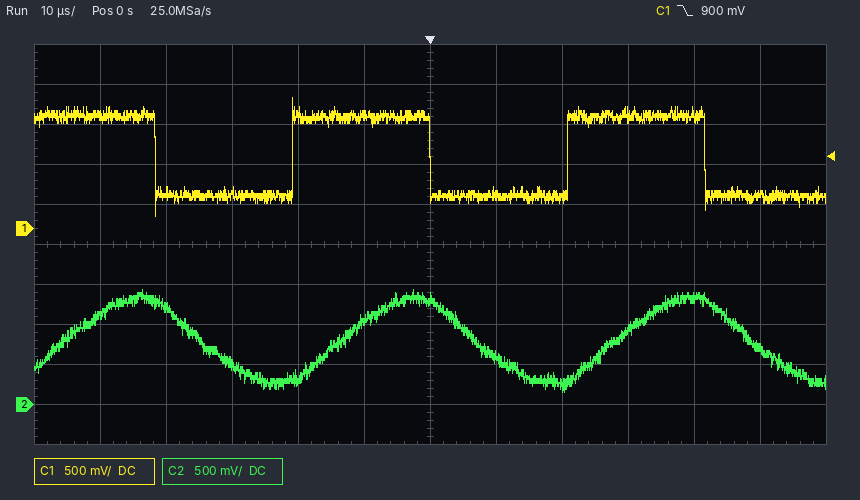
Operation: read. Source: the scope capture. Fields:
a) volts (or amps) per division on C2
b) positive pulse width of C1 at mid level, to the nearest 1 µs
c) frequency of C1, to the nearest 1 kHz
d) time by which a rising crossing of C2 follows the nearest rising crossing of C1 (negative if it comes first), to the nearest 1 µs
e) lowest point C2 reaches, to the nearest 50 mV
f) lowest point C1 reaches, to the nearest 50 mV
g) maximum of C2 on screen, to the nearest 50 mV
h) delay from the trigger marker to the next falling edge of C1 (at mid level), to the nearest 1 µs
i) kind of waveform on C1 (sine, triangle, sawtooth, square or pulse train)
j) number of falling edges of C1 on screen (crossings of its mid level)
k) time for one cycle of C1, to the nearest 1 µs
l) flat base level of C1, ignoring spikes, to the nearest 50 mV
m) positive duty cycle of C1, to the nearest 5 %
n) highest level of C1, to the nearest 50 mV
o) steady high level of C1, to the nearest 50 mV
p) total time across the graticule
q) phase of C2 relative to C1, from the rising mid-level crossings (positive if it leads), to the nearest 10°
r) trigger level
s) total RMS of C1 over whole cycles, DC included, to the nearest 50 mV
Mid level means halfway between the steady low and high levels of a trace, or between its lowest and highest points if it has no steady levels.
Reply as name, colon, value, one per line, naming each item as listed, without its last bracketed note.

volts (or amps) per division on C2: 500 mV
positive pulse width of C1 at mid level, to the nearest 1 µs: 21 µs
frequency of C1, to the nearest 1 kHz: 24 kHz
time by which a rising crossing of C2 follows the nearest rising crossing of C1 (negative if it comes first), to the nearest 1 µs: +7 µs
lowest point C2 reaches, to the nearest 50 mV: 150 mV
lowest point C1 reaches, to the nearest 50 mV: 150 mV
maximum of C2 on screen, to the nearest 50 mV: 1.45 V
delay from the trigger marker to the next falling edge of C1 (at mid level), to the nearest 1 µs: 42 µs
kind of waveform on C1: square
number of falling edges of C1 on screen: 3
time for one cycle of C1, to the nearest 1 µs: 42 µs
flat base level of C1, ignoring spikes, to the nearest 50 mV: 400 mV
positive duty cycle of C1, to the nearest 5 %: 50 %
highest level of C1, to the nearest 50 mV: 1.65 V
steady high level of C1, to the nearest 50 mV: 1.40 V
total time across the graticule: 120 µs
phase of C2 relative to C1, from the rising mid-level crossings (positive if it leads), to the nearest 10°: -60°
trigger level: 900 mV
total RMS of C1 over whole cycles, DC included, to the nearest 50 mV: 1.05 V
